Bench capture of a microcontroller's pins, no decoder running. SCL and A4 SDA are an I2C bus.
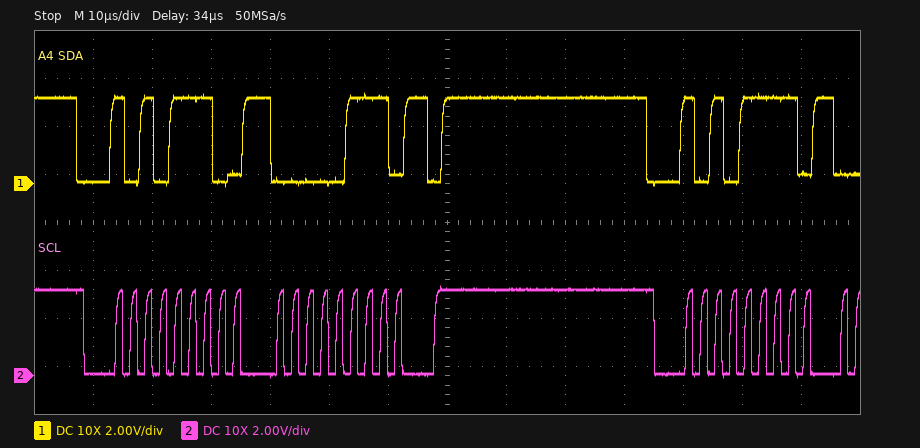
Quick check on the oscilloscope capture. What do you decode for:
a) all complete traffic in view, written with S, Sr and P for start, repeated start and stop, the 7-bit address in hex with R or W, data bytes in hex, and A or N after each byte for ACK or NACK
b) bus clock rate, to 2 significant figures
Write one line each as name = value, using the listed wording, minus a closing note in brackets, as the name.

all complete traffic in view, written with S, Sr and P for start, repeated start and stop, the 7-bit address in hex with R or W, data bytes in hex, and A or N after each byte for ACK or NACK = S 57W A 07 A P S 57R A
bus clock rate, to 2 significant figures = 400 kHz
